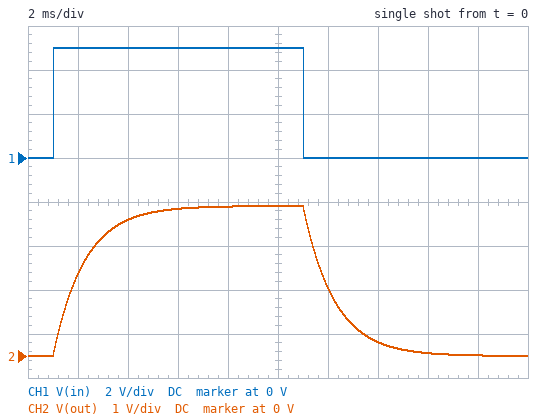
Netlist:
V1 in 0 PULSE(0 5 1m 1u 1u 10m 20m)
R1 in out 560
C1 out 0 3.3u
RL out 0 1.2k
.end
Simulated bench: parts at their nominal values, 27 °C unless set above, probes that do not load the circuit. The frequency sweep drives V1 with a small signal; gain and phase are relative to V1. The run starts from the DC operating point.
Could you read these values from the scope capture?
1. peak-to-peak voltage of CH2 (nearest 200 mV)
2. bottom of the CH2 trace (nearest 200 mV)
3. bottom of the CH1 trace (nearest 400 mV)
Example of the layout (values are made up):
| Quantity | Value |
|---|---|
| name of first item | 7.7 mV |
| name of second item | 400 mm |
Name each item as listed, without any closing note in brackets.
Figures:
| Quantity | Value |
|---|---|
| peak-to-peak voltage of CH2 | 3.4 V |
| bottom of the CH2 trace | 0 V |
| bottom of the CH1 trace | 0 V |
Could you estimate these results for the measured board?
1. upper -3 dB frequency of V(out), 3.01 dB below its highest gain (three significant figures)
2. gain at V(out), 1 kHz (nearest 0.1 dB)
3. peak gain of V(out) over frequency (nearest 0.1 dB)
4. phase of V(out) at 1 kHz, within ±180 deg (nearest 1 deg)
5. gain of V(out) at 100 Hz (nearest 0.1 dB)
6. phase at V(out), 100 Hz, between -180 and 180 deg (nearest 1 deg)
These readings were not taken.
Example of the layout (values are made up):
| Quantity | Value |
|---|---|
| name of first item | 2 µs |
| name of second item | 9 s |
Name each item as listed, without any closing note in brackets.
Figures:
| Quantity | Value |
|---|---|
| upper -3 dB frequency of V(out), 3.01 dB below its highest gain | 126 Hz |
| gain at V(out), 1 kHz | -21.4 dB |
| peak gain of V(out) over frequency | -3.3 dB |
| phase of V(out) at 1 kHz, within ±180 deg | -83 deg |
| gain of V(out) at 100 Hz | -5.4 dB |
| phase at V(out), 100 Hz, between -180 and 180 deg | -38 deg |
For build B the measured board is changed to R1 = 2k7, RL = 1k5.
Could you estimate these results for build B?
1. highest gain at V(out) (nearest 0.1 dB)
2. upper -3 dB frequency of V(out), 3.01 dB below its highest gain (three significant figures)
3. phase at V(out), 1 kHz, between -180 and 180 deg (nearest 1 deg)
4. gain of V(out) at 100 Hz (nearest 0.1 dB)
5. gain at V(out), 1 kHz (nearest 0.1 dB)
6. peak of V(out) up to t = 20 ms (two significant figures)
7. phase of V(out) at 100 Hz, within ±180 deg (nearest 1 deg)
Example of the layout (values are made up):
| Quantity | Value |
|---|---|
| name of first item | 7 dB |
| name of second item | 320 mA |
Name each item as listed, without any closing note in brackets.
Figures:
| Quantity | Value |
|---|---|
| highest gain at V(out) | -8.9 dB |
| upper -3 dB frequency of V(out), 3.01 dB below its highest gain | 50.0 Hz |
| phase at V(out), 1 kHz, between -180 and 180 deg | -87 deg |
| gain of V(out) at 100 Hz | -15.9 dB |
| gain at V(out), 1 kHz | -35.0 dB |
| peak of V(out) up to t = 20 ms | 1.7 V |
| phase of V(out) at 100 Hz, within ±180 deg | -63 deg |
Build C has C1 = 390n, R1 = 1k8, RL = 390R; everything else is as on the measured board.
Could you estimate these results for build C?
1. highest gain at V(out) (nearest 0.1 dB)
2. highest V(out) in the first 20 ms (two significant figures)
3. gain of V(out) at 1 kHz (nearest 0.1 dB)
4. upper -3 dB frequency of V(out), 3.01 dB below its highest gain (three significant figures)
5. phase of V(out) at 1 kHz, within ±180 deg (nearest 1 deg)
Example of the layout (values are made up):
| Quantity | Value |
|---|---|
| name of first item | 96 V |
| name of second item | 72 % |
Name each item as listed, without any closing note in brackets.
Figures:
| Quantity | Value |
|---|---|
| highest gain at V(out) | -15.0 dB |
| highest V(out) in the first 20 ms | 890 mV |
| gain of V(out) at 1 kHz | -17.1 dB |
| upper -3 dB frequency of V(out), 3.01 dB below its highest gain | 1.27 kHz |
| phase of V(out) at 1 kHz, within ±180 deg | -38 deg |
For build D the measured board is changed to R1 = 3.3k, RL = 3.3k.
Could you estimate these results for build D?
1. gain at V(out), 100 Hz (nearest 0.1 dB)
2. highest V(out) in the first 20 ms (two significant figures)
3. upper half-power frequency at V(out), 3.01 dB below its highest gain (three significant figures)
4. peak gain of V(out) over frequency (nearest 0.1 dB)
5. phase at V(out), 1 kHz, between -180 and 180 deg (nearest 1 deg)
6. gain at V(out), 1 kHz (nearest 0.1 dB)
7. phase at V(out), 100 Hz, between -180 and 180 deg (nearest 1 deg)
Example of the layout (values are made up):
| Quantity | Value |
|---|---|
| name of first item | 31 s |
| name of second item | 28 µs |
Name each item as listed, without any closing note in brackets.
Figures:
| Quantity | Value |
|---|---|
| gain at V(out), 100 Hz | -17.1 dB |
| highest V(out) in the first 20 ms | 2.1 V |
| upper half-power frequency at V(out), 3.01 dB below its highest gain | 29.2 Hz |
| peak gain of V(out) over frequency | -6.0 dB |
| phase at V(out), 1 kHz, between -180 and 180 deg | -88 deg |
| gain at V(out), 1 kHz | -36.7 dB |
| phase at V(out), 100 Hz, between -180 and 180 deg | -74 deg |
